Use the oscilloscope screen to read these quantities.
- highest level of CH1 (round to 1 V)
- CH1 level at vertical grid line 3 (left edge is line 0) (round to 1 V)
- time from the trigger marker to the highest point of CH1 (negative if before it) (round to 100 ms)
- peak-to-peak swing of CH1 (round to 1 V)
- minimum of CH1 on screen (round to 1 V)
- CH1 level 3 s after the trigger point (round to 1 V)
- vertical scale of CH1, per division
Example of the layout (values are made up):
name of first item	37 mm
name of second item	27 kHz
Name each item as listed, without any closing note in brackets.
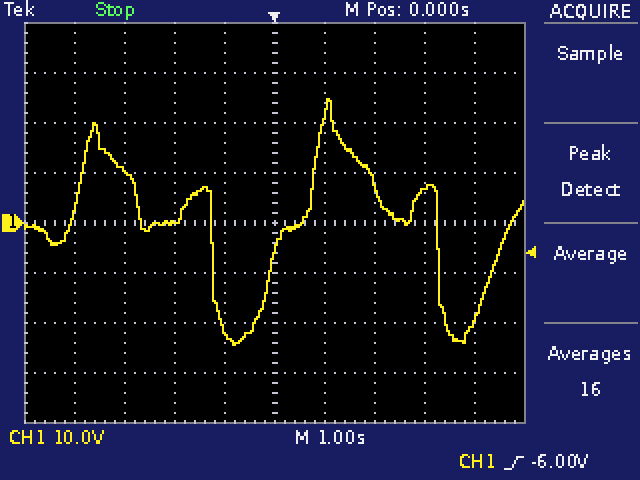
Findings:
highest level of CH1	25 V
CH1 level at vertical grid line 3 (left edge is line 0)	0 V
time from the trigger marker to the highest point of CH1 (negative if before it)	+1.1 s
peak-to-peak swing of CH1	49 V
minimum of CH1 on screen	-24 V
CH1 level 3 s after the trigger point	7 V
vertical scale of CH1, per division	10 V
